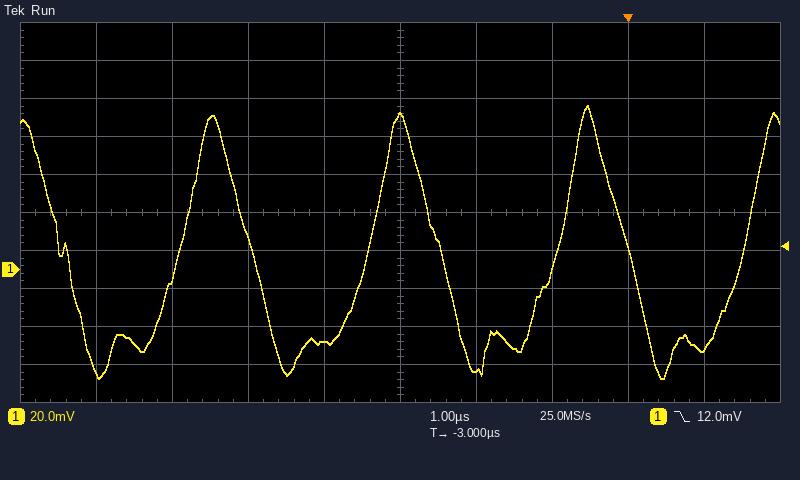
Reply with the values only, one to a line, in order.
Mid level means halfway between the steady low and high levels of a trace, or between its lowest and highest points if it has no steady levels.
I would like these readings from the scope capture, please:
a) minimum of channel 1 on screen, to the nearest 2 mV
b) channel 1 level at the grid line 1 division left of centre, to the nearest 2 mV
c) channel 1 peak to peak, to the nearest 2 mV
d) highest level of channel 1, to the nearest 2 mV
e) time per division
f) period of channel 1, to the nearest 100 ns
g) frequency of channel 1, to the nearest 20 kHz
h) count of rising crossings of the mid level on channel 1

-58 mV
-38 mV
144 mV
86 mV
1 µs
2.5 µs
400 kHz
4
